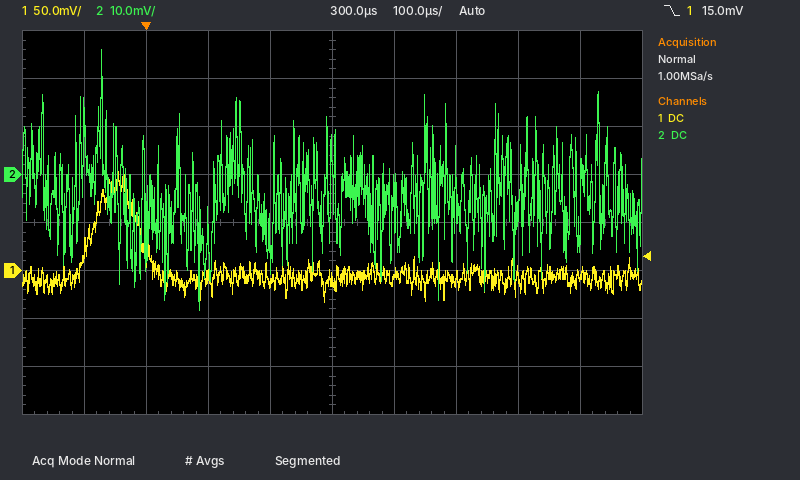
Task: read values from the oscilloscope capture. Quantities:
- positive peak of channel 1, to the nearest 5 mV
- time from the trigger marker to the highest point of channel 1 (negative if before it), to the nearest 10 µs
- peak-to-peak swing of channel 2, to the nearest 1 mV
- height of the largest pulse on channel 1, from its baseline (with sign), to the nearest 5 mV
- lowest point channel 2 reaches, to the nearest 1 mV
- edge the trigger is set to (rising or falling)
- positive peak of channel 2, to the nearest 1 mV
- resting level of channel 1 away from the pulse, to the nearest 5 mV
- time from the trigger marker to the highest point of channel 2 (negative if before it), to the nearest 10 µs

105 mV
-40 µs
54 mV
+110 mV
-28 mV
falling
26 mV
-5 mV
-70 µs
